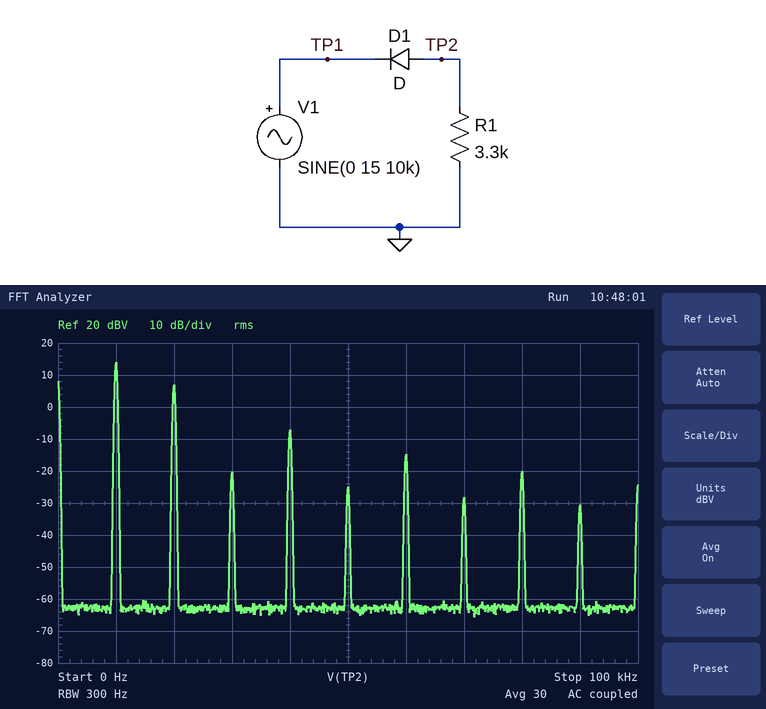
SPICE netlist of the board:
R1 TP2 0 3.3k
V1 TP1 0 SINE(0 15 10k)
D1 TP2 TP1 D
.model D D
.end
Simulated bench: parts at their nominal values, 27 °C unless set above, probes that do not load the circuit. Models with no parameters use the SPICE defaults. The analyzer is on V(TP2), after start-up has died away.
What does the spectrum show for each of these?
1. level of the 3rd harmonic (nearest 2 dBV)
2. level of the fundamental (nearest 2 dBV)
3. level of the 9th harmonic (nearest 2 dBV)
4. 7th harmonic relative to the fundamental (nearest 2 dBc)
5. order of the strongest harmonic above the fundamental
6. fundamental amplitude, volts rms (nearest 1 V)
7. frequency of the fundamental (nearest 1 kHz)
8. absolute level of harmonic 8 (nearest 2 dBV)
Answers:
-20 dBV
14 dBV
-30 dBV
-42 dBc
2
5 V
10 kHz
-20 dBV
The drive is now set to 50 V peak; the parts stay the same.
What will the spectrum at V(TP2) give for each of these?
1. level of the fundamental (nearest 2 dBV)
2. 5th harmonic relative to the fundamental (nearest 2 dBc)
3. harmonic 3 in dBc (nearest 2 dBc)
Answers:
24 dBV
-50 dBc
-44 dBc
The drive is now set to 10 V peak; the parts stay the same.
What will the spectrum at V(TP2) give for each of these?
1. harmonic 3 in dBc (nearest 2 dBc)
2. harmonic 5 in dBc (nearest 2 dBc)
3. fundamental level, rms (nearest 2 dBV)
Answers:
-30 dBc
-36 dBc
10 dBV
